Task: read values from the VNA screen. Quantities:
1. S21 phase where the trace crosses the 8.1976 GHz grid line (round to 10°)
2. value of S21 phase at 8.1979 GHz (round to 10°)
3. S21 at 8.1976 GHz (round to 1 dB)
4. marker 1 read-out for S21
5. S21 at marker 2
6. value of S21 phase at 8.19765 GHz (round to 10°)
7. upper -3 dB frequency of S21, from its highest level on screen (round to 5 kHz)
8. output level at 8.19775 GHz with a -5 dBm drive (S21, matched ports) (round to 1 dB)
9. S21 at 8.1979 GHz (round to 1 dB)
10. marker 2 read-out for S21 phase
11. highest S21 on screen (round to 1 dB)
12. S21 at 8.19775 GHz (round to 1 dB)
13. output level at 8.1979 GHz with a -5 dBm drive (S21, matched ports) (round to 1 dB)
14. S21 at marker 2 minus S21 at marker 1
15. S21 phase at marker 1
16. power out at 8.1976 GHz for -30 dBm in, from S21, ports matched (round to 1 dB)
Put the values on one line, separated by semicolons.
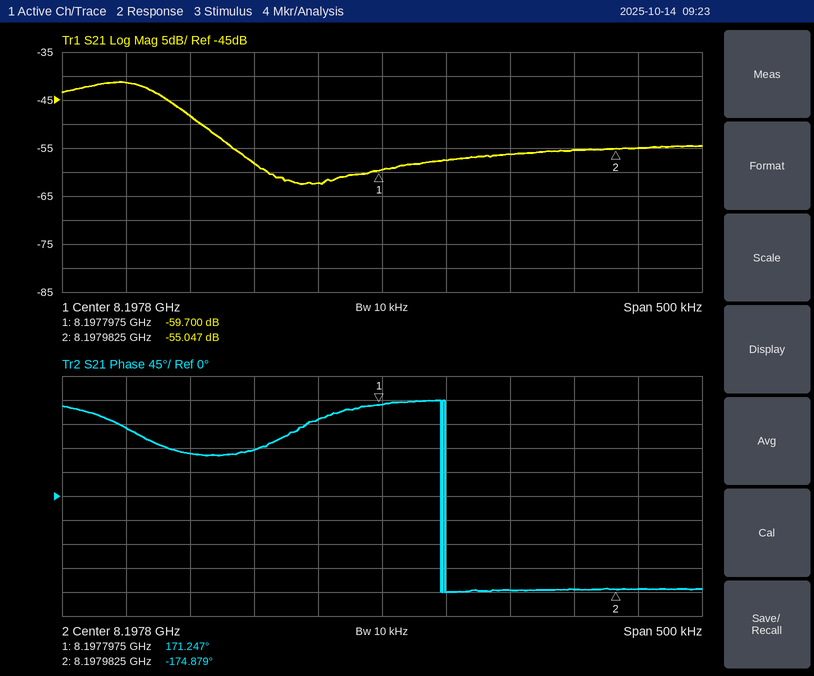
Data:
130°; -180°; -41 dB; -59.700 dB; -55.047 dB; 80°; 8.197630 GHz; -67 dBm; -56 dB; -174.879°; -41 dB; -62 dB; -61 dBm; 4.653 dB; 171.247°; -71 dBm
